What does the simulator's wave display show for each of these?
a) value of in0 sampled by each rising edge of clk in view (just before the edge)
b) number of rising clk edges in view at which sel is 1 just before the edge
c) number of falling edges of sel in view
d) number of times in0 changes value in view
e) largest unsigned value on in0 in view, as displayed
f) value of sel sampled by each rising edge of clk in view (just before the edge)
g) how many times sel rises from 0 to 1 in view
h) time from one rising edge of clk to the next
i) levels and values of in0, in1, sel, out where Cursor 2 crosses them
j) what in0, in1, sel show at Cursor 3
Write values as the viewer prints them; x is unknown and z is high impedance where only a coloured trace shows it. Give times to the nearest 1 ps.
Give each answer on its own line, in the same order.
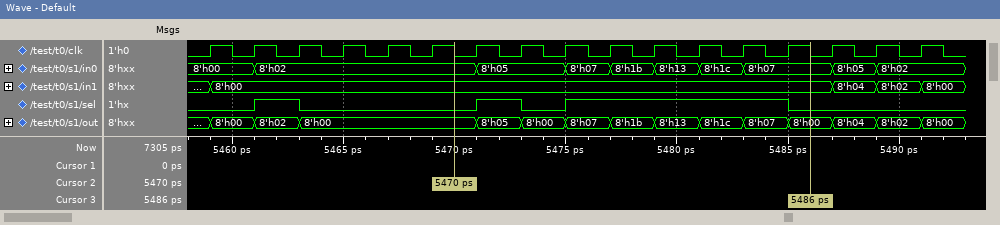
8'h00, 8'h00, 8'h02, 8'h02, 8'h02, 8'h02, 8'h02, 8'h05, 8'h05, 8'h07, 8'h1b, 8'h13, 8'h1c, 8'h07, 8'h07, 8'h05, 8'h02
7
3
9
8'h1c
0 0 1 0 0 0 0 1 0 1 1 1 1 1 0 0 0
3
2 ps
in0=8'h02, in1=8'h00, sel=0, out=8'h00
in0=8'h07, in1=8'h00, sel=0
